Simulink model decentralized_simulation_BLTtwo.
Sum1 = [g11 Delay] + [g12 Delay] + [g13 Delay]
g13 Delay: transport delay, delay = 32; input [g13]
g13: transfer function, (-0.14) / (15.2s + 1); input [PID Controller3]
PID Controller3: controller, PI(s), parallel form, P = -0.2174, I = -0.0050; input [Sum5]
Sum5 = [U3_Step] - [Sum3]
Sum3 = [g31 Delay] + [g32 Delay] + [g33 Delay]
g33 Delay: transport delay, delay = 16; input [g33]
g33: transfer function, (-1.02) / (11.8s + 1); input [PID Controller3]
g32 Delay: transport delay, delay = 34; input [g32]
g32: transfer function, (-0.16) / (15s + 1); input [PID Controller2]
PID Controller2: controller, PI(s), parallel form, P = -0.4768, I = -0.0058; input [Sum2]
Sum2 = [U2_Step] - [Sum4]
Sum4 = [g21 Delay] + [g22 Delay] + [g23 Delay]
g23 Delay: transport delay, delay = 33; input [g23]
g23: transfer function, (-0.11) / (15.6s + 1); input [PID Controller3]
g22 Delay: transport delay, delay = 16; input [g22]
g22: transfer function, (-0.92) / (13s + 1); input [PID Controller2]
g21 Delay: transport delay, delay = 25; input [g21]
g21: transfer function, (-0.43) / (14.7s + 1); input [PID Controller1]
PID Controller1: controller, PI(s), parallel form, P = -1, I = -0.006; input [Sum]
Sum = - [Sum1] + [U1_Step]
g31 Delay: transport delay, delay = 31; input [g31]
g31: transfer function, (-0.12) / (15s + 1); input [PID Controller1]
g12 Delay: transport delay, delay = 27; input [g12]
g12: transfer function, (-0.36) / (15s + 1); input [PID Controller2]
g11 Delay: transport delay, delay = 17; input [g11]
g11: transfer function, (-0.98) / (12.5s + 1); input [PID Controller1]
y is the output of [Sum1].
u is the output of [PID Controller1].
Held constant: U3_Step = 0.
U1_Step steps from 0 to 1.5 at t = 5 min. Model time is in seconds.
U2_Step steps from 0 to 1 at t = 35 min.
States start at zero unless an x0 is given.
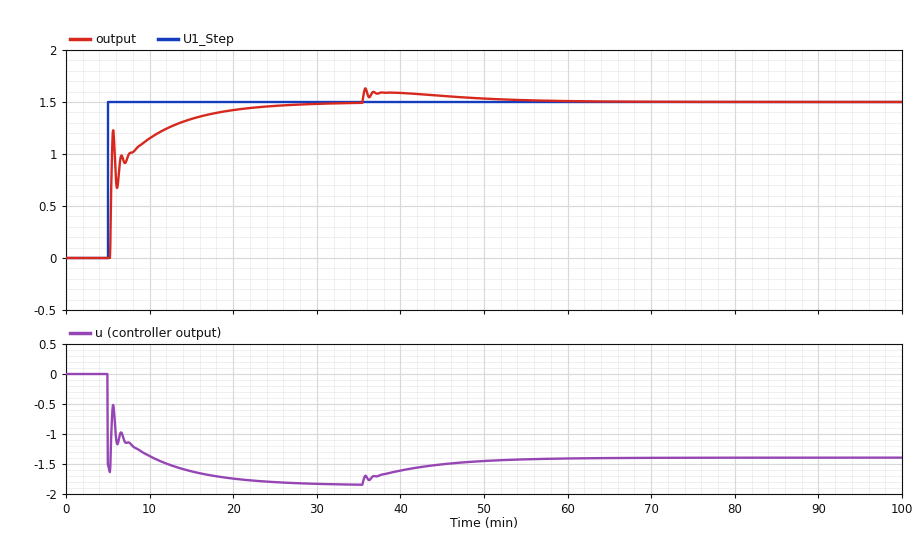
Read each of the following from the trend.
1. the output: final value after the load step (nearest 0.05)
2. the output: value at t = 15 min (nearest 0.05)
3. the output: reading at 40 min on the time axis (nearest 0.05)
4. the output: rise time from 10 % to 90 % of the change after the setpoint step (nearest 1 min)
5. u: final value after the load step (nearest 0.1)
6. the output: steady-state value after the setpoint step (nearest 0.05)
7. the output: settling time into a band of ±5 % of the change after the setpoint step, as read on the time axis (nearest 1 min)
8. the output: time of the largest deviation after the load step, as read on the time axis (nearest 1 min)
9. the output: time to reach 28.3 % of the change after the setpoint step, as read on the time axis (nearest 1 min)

1.50
1.35
1.60
10 min
-1.4
1.50
20 min
36 min
5 min
